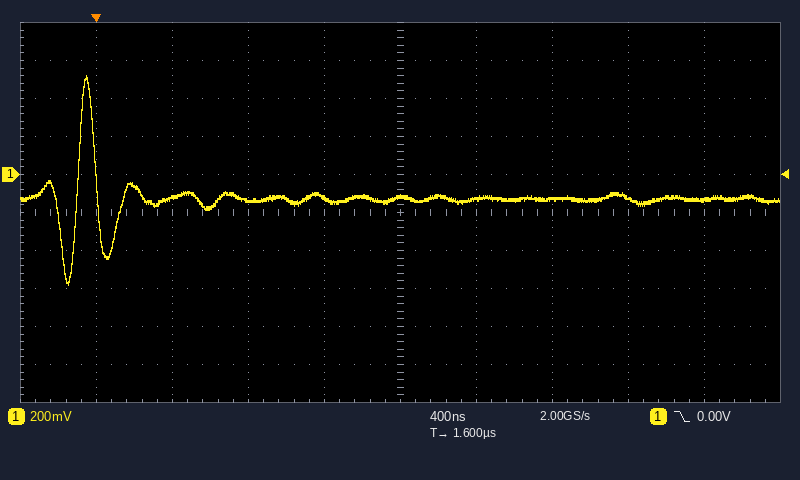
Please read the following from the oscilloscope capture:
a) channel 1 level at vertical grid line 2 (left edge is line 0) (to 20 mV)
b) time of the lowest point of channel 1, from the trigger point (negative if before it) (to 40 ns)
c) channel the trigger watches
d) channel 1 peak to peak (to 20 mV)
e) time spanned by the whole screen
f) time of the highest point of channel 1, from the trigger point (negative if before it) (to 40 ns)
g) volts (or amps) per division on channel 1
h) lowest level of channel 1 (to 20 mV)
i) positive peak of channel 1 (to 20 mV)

-120 mV
-160 ns
channel 1
1.10 V
4 µs
-40 ns
200 mV
-580 mV
520 mV
